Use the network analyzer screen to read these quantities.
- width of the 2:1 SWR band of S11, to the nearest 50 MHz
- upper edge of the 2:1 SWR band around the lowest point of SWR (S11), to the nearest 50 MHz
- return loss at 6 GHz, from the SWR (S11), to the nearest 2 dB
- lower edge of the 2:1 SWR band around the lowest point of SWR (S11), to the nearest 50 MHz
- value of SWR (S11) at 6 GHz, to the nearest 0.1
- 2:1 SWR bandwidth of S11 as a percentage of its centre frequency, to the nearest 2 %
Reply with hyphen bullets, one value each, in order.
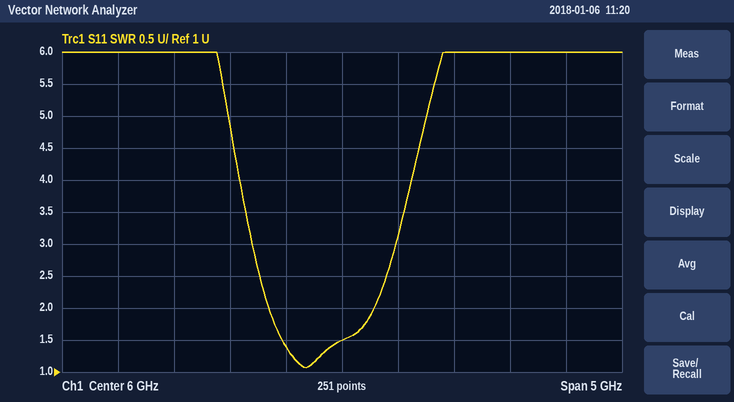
- 950 MHz
- 6.30 GHz
- 14 dB
- 5.35 GHz
- 1.5
- 16 %
